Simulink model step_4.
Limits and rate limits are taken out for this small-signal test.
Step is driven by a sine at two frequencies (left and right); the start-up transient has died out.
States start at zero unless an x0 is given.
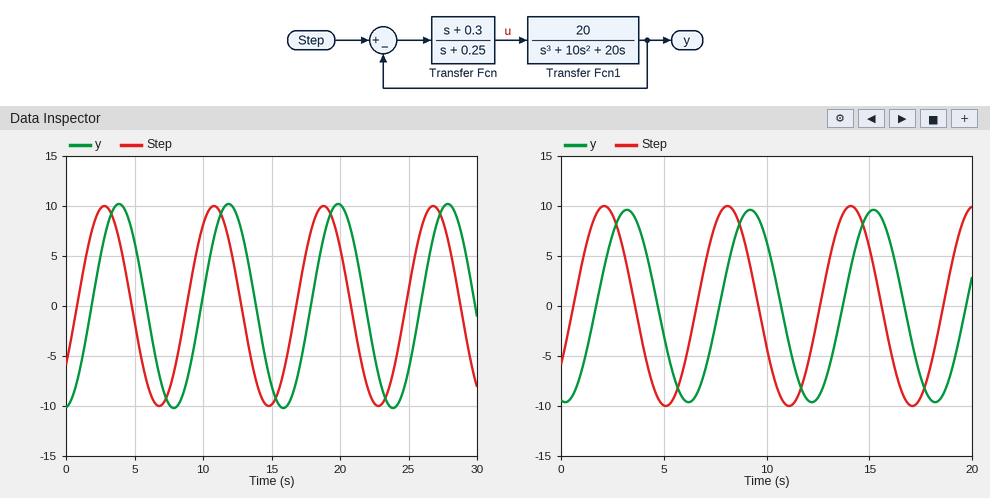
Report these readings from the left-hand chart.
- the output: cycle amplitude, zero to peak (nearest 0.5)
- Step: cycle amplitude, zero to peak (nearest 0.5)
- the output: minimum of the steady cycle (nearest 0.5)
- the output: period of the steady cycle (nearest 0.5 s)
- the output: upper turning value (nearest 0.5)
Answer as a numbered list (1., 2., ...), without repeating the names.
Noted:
1. 10.0
2. 10.0
3. -10.0
4. 8.0 s
5. 10.0
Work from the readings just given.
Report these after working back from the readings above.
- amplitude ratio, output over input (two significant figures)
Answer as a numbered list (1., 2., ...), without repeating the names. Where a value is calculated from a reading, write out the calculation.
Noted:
1. 10 / 10 = 1.0
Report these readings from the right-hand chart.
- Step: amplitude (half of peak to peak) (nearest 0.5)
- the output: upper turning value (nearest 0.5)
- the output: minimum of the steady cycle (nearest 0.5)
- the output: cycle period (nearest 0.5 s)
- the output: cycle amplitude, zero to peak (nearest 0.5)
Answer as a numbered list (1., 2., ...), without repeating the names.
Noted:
1. 10.0
2. 9.5
3. -9.5
4. 6.0 s
5. 9.5
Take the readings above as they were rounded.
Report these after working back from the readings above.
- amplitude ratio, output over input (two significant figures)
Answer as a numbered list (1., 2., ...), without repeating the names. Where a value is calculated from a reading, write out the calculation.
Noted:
1. 9.5 / 10 = 0.95
